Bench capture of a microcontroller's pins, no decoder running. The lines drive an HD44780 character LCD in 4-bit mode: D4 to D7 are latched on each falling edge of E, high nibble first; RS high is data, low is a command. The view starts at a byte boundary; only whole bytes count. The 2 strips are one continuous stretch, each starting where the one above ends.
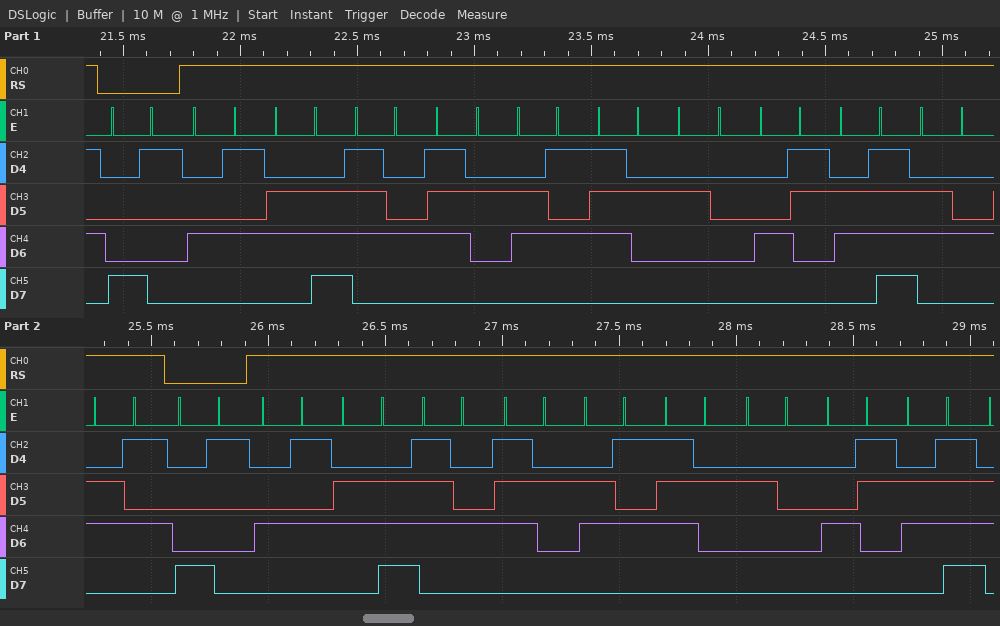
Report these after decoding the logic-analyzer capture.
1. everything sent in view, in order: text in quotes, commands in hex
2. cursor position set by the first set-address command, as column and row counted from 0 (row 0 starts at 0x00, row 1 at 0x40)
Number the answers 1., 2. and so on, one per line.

1. 0x81 "Entrer Code" 0x81 "Entrer Co"
2. column 1, row 0
